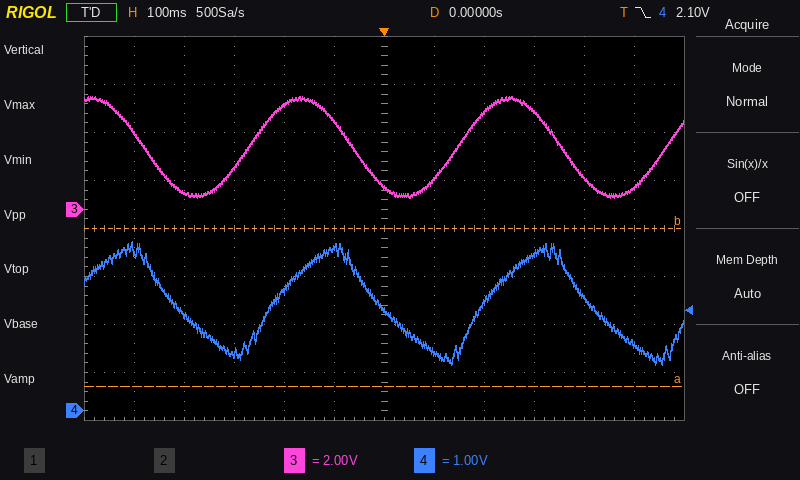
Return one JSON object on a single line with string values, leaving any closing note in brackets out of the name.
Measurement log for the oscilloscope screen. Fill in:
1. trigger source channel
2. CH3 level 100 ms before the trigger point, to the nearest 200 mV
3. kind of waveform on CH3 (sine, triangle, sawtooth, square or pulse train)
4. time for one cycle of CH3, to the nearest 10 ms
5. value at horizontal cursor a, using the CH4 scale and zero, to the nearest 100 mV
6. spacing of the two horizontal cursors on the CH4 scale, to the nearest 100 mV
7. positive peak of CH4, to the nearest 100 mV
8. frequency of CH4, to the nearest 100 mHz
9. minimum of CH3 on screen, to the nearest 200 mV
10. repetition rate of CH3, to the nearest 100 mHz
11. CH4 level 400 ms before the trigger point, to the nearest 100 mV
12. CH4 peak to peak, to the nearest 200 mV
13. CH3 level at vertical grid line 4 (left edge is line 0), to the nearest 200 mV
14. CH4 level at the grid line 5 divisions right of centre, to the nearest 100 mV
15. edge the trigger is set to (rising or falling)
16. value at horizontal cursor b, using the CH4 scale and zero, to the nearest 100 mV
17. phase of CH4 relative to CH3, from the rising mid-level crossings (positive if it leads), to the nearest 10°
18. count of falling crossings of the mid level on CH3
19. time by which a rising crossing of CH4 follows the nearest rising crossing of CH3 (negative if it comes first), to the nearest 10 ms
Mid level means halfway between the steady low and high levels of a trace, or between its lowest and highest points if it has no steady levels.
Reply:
{"trigger source channel": "CH4", "CH3 level 100 ms before the trigger point, to the nearest 200 mV": "3.6 V", "kind of waveform on CH3": "sine", "time for one cycle of CH3, to the nearest 10 ms": "420 ms", "value at horizontal cursor a, using the CH4 scale and zero, to the nearest 100 mV": "500 mV", "spacing of the two horizontal cursors on the CH4 scale, to the nearest 100 mV": "3.3 V", "positive peak of CH4, to the nearest 100 mV": "3.5 V", "frequency of CH4, to the nearest 100 mHz": "2.4 Hz", "minimum of CH3 on screen, to the nearest 200 mV": "400 mV", "repetition rate of CH3, to the nearest 100 mHz": "2.4 Hz", "CH4 level 400 ms before the trigger point, to the nearest 100 mV": "2.0 V", "CH4 peak to peak, to the nearest 200 mV": "2.6 V", "CH3 level at vertical grid line 4 (left edge is line 0), to the nearest 200 mV": "4.4 V", "CH4 level at the grid line 5 divisions right of centre, to the nearest 100 mV": "1.4 V", "edge the trigger is set to": "falling", "value at horizontal cursor b, using the CH4 scale and zero, to the nearest 100 mV": "3.8 V", "phase of CH4 relative to CH3, from the rising mid-level crossings (positive if it leads), to the nearest 10°": "-40°", "count of falling crossings of the mid level on CH3": "3", "time by which a rising crossing of CH4 follows the nearest rising crossing of CH3 (negative if it comes first), to the nearest 10 ms": "+50 ms"}
